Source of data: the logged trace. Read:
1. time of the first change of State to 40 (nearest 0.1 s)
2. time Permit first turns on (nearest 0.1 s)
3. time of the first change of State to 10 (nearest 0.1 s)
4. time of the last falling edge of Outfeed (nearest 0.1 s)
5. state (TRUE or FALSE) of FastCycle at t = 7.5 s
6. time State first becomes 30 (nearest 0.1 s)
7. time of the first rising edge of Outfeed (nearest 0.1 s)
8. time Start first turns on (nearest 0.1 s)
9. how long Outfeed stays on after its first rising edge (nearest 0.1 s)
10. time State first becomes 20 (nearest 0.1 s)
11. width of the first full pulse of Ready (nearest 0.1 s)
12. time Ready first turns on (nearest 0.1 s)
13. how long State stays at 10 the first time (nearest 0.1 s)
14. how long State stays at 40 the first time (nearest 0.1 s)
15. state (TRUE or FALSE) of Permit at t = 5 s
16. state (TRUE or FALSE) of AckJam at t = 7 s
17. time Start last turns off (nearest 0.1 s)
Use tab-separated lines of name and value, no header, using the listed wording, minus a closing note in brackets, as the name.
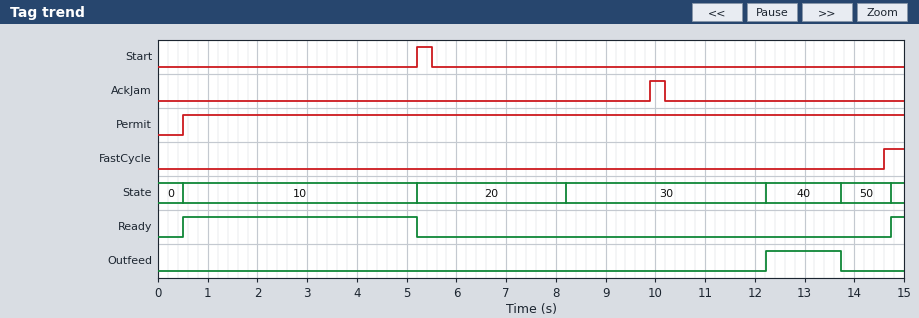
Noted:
time of the first change of State to 40	12.2 s
time Permit first turns on	0.5 s
time of the first change of State to 10	0.5 s
time of the last falling edge of Outfeed	13.7 s
state (TRUE or FALSE) of FastCycle at t = 7.5 s	FALSE
time State first becomes 30	8.2 s
time of the first rising edge of Outfeed	12.2 s
time Start first turns on	5.2 s
how long Outfeed stays on after its first rising edge	1.5 s
time State first becomes 20	5.2 s
width of the first full pulse of Ready	4.7 s
time Ready first turns on	0.5 s
how long State stays at 10 the first time	4.7 s
how long State stays at 40 the first time	1.5 s
state (TRUE or FALSE) of Permit at t = 5 s	TRUE
state (TRUE or FALSE) of AckJam at t = 7 s	FALSE
time Start last turns off	5.5 s
